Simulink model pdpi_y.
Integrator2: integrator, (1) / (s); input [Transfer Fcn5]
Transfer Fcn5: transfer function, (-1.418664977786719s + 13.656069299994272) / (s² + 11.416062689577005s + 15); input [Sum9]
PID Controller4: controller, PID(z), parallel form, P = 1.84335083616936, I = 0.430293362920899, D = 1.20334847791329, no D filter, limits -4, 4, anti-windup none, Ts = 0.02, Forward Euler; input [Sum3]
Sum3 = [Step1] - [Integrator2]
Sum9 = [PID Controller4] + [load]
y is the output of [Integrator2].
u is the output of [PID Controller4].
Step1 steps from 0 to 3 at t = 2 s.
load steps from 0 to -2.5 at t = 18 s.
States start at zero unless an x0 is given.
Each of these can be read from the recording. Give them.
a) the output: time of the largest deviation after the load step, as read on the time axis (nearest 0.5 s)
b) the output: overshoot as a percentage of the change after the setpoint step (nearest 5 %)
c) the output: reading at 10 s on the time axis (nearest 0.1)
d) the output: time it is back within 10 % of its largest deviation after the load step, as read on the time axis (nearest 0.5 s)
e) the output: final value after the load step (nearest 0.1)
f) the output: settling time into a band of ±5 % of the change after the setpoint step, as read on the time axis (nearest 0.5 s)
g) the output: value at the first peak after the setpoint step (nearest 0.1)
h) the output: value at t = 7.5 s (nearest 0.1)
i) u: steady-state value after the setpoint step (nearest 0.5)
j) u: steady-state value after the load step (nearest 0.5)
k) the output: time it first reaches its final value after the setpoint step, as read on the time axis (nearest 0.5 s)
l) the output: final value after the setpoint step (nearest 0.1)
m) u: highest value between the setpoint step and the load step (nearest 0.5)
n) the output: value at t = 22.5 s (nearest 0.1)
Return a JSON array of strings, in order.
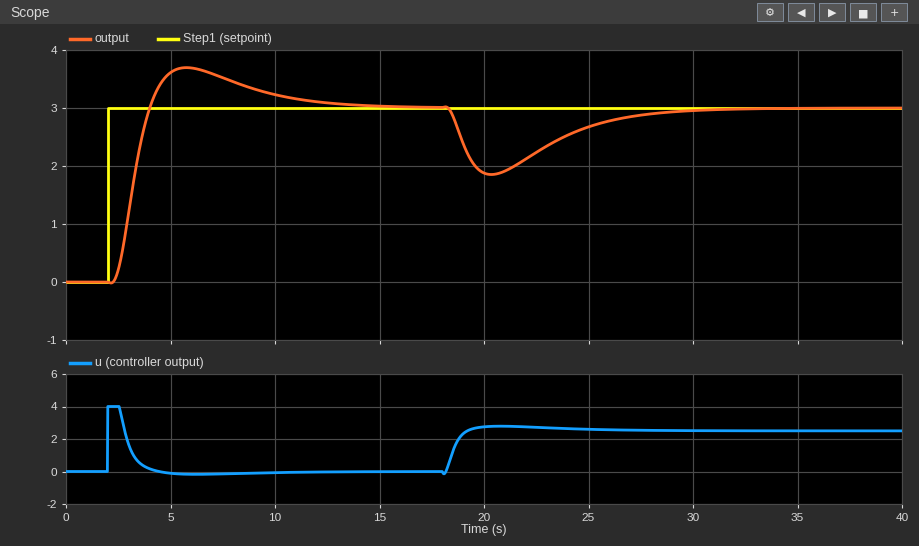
["20.5 s", "25 %", "3.2", "27.5 s", "3.0", "11.0 s", "3.7", "3.5", "0.0", "2.5", "4.0 s", "3.0", "4.0", "2.2"]
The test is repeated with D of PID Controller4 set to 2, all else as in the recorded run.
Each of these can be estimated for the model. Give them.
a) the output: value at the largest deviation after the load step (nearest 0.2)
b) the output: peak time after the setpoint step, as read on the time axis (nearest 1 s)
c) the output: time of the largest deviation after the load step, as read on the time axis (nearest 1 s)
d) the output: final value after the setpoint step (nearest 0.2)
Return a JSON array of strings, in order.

["2.0", "7 s", "21 s", "3.0"]
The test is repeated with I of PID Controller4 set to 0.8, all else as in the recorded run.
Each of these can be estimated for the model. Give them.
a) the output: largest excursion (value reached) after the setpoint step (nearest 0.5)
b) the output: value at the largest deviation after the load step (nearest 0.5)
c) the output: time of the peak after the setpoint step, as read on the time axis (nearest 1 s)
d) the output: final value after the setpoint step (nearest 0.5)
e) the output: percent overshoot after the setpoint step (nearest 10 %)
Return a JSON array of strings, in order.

["4.0", "2.0", "5 s", "3.0", "40 %"]
